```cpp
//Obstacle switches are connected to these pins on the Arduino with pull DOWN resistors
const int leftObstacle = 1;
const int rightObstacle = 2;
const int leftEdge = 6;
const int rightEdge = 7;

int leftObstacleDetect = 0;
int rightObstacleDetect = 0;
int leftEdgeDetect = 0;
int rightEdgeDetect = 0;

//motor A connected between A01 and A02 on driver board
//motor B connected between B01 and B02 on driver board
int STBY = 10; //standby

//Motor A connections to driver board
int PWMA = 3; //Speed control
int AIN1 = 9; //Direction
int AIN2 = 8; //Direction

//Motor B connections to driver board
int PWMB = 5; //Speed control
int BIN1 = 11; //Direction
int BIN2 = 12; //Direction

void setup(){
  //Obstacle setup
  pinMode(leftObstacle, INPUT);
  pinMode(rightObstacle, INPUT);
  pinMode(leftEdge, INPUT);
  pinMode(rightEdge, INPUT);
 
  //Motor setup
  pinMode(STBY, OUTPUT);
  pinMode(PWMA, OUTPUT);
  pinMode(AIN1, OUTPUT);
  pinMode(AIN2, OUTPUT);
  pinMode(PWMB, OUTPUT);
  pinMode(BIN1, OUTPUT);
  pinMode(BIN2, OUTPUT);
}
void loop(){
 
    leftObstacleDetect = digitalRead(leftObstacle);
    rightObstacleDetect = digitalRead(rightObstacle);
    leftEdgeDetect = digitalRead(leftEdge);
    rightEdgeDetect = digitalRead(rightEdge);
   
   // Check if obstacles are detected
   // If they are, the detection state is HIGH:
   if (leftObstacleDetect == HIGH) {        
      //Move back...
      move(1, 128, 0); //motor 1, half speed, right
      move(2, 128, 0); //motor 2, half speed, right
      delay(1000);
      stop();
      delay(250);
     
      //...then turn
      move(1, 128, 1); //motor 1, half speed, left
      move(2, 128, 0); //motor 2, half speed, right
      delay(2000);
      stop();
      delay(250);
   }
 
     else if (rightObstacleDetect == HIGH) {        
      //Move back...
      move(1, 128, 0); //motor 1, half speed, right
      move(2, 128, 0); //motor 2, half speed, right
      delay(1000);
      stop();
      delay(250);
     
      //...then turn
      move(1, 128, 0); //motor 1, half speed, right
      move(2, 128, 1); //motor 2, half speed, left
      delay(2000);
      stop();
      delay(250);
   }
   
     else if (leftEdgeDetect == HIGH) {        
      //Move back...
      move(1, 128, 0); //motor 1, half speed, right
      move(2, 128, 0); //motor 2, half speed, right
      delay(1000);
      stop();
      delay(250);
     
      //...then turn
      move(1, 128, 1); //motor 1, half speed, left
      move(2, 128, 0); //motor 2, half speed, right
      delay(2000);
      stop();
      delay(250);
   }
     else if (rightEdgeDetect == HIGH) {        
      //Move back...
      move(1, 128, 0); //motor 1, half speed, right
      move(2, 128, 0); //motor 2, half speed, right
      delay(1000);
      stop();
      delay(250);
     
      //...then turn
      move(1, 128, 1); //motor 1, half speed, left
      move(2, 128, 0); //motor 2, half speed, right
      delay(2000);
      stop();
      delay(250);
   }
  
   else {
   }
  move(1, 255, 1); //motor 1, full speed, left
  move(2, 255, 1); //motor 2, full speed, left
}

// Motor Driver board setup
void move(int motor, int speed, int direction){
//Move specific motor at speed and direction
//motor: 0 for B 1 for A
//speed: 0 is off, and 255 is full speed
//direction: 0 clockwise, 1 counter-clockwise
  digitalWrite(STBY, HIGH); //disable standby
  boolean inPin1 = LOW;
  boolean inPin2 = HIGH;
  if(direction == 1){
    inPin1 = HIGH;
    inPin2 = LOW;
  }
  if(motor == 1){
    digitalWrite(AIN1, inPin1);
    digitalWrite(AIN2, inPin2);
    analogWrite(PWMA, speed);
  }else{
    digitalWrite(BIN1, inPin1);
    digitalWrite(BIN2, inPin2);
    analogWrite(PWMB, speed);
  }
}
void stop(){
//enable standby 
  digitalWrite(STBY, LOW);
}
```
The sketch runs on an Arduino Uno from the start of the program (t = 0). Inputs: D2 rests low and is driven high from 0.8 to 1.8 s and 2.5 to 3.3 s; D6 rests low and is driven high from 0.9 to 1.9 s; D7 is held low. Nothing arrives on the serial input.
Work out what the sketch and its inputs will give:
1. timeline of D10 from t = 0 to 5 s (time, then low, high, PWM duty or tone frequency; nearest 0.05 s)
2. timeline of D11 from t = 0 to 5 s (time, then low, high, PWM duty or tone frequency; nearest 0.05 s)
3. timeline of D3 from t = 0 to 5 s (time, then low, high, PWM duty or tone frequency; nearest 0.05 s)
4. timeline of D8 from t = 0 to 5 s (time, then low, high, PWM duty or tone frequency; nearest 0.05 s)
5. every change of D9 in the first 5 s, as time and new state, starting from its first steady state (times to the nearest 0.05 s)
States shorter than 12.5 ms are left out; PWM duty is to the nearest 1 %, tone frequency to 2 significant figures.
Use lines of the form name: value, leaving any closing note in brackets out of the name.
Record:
timeline of D10 from t = 0 to 5 s: 0 s high; 1.8 s low; 2.05 s high; 4.05 s low; 4.3 s high
timeline of D11 from t = 0 to 5 s: 0 s high; 0.8 s low; 2.05 s high
timeline of D3 from t = 0 to 5 s: 0 s high; 0.8 s PWM 50 %; 4.3 s high
timeline of D8 from t = 0 to 5 s: 0 s low; 0.8 s high; 4.3 s low
every change of D9 in the first 5 s, as time and new state, starting from its first steady state: 0 s high; 0.8 s low; 4.3 s high
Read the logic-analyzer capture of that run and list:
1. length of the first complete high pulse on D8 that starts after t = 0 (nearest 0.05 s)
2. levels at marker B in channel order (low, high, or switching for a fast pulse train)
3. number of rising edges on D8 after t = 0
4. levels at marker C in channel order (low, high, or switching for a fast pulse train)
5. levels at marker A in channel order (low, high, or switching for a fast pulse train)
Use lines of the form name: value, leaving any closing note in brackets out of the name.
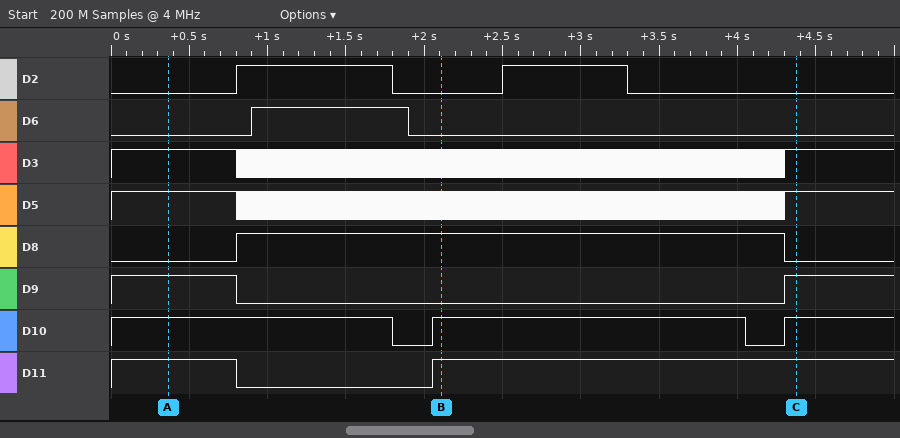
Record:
length of the first complete high pulse on D8 that starts after t = 0: 3.50 s
levels at marker B in channel order: D2 low, D6 low, D3 switching, D5 switching, D8 high, D9 low, D10 high, D11 high
number of rising edges on D8 after t = 0: 1
levels at marker C in channel order: D2 low, D6 low, D3 high, D5 high, D8 low, D9 high, D10 high, D11 high
levels at marker A in channel order: D2 low, D6 low, D3 high, D5 high, D8 low, D9 high, D10 high, D11 high
